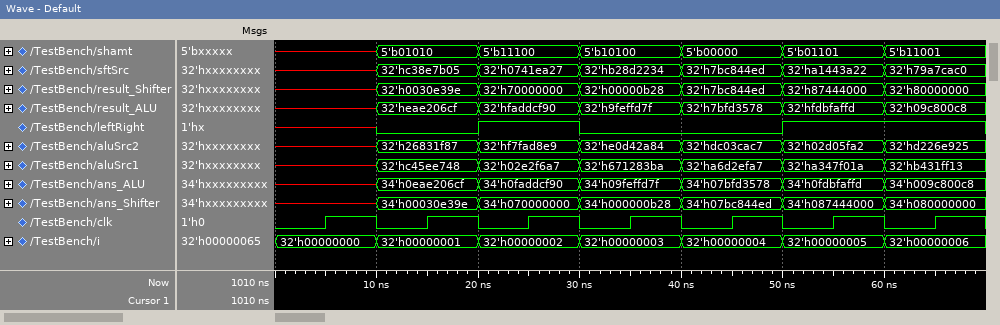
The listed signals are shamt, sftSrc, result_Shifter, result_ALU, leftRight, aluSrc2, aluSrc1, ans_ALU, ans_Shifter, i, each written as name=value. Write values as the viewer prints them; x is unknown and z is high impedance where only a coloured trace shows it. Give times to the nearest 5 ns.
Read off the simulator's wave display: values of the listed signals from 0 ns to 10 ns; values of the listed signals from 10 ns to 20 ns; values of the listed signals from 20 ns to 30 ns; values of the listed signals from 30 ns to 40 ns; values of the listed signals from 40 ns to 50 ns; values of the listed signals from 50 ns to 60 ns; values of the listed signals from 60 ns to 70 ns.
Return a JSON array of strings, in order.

["shamt=x, sftSrc=x, result_Shifter=x, result_ALU=x, leftRight=x, aluSrc2=x, aluSrc1=x, ans_ALU=x, ans_Shifter=x, i=32'h00000000", "shamt=5'b01010, sftSrc=32'hc38e7b05, result_Shifter=32'h0030e39e, result_ALU=32'heae206cf, leftRight=0, aluSrc2=32'h26831f87, aluSrc1=32'hc45ee748, ans_ALU=34'h0eae206cf, ans_Shifter=34'h00030e39e, i=32'h00000001", "shamt=5'b11100, sftSrc=32'h0741ea27, result_Shifter=32'h70000000, result_ALU=32'hfaddcf90, leftRight=1, aluSrc2=32'hf7fad8e9, aluSrc1=32'h02e2f6a7, ans_ALU=34'h0faddcf90, ans_Shifter=34'h070000000, i=32'h00000002", "shamt=5'b10100, sftSrc=32'hb28d2234, result_Shifter=32'h00000b28, result_ALU=32'h9feffd7f, leftRight=0, aluSrc2=32'he0d42a84, aluSrc1=32'h671283ba, ans_ALU=34'h09feffd7f, ans_Shifter=34'h000000b28, i=32'h00000003", "shamt=5'b00000, sftSrc=32'h7bc844ed, result_Shifter=32'h7bc844ed, result_ALU=32'h7bfd3578, leftRight=0, aluSrc2=32'hdc03cac7, aluSrc1=32'ha6d2efa7, ans_ALU=34'h07bfd3578, ans_Shifter=34'h07bc844ed, i=32'h00000004", "shamt=5'b01101, sftSrc=32'ha1443a22, result_Shifter=32'h87444000, result_ALU=32'hfdbfaffd, leftRight=1, aluSrc2=32'h02d05fa2, aluSrc1=32'ha347f01a, ans_ALU=34'h0fdbfaffd, ans_Shifter=34'h087444000, i=32'h00000005", "shamt=5'b11001, sftSrc=32'h79a7cac0, result_Shifter=32'h80000000, result_ALU=32'h09c800c8, leftRight=1, aluSrc2=32'hd226e925, aluSrc1=32'hb431ff13, ans_ALU=34'h009c800c8, ans_Shifter=34'h080000000, i=32'h00000006"]
